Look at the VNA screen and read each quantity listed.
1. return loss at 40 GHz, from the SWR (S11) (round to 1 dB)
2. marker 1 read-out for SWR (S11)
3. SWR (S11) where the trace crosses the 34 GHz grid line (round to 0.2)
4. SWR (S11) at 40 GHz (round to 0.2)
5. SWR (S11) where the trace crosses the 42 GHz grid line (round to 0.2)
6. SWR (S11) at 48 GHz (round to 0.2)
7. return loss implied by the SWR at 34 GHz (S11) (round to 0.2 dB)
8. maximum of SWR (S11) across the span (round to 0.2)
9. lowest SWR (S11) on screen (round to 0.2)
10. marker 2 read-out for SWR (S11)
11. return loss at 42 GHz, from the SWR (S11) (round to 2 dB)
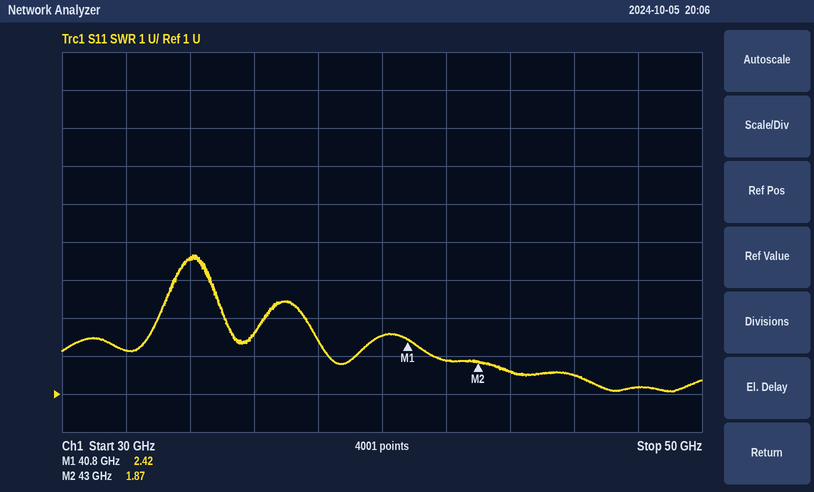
7 dB
2.42
4.6
2.6
1.8
1.2
3.8 dB
4.6
1.0
1.87
10 dB
